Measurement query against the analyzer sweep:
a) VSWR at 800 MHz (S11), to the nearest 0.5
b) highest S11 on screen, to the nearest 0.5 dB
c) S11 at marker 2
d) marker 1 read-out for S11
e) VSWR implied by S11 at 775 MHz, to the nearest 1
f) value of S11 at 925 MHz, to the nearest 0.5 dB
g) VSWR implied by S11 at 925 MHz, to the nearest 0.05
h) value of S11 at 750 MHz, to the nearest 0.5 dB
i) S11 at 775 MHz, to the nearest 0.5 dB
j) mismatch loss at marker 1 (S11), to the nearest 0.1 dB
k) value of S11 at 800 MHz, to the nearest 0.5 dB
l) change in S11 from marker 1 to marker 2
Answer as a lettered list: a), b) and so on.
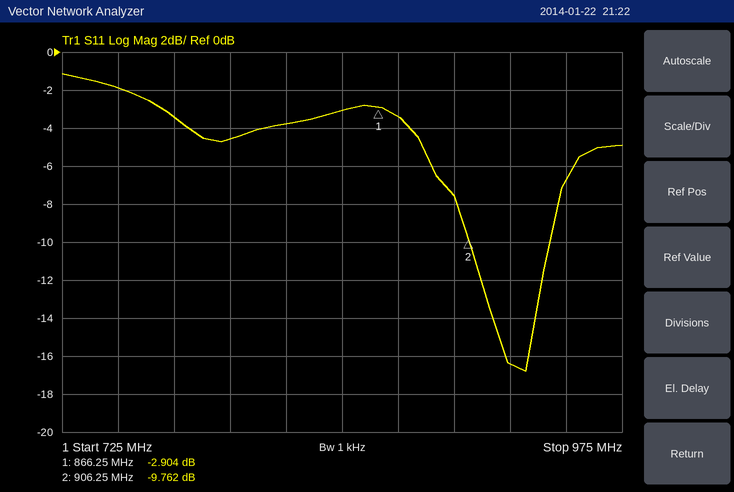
a) 4.0
b) -1.0 dB
c) -9.762 dB
d) -2.904 dB
e) 5
f) -16.5 dB
g) 1.35
h) -2.0 dB
i) -3.5 dB
j) 3.1 dB
k) -4.5 dB
l) -6.858 dB
